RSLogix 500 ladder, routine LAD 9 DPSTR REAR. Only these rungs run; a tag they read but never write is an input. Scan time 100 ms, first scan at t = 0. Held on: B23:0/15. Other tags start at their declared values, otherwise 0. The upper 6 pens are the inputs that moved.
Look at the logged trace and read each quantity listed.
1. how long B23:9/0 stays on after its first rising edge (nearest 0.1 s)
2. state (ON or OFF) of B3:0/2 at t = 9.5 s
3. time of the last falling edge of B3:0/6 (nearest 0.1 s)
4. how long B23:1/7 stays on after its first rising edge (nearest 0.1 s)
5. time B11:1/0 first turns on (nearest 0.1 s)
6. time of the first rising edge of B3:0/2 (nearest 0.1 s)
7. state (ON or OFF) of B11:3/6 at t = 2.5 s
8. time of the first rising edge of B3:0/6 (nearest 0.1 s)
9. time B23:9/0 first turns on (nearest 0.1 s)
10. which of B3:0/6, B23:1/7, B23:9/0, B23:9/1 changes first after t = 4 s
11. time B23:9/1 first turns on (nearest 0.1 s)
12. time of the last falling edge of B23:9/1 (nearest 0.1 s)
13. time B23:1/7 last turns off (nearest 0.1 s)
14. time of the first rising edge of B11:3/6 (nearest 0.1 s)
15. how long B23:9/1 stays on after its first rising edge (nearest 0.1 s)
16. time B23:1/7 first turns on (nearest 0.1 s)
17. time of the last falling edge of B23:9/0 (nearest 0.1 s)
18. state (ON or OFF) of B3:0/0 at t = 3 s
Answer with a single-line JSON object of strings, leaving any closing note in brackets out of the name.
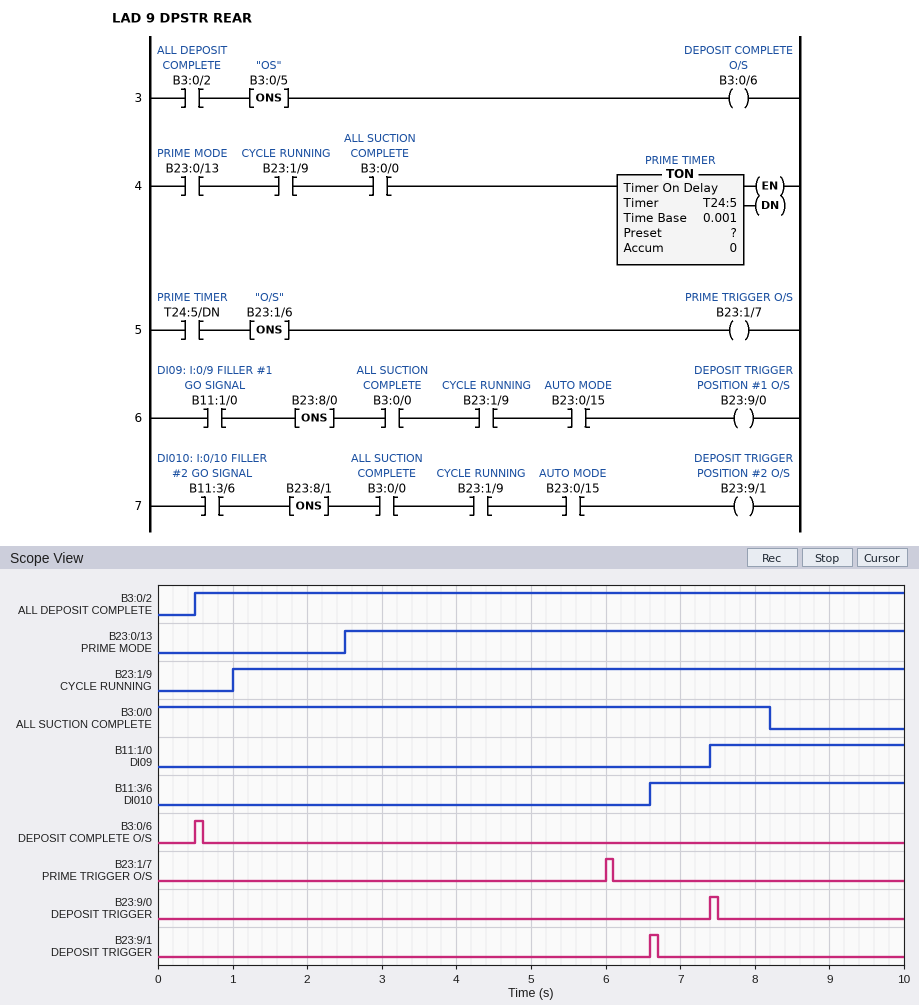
{"how long B23:9/0 stays on after its first rising edge": "0.1 s", "state (ON or OFF) of B3:0/2 at t = 9.5 s": "ON", "time of the last falling edge of B3:0/6": "0.6 s", "how long B23:1/7 stays on after its first rising edge": "0.1 s", "time B11:1/0 first turns on": "7.4 s", "time of the first rising edge of B3:0/2": "0.5 s", "state (ON or OFF) of B11:3/6 at t = 2.5 s": "OFF", "time of the first rising edge of B3:0/6": "0.5 s", "time B23:9/0 first turns on": "7.4 s", "which of B3:0/6, B23:1/7, B23:9/0, B23:9/1 changes first after t = 4 s": "B23:1/7", "time B23:9/1 first turns on": "6.6 s", "time of the last falling edge of B23:9/1": "6.7 s", "time B23:1/7 last turns off": "6.1 s", "time of the first rising edge of B11:3/6": "6.6 s", "how long B23:9/1 stays on after its first rising edge": "0.1 s", "time B23:1/7 first turns on": "6.0 s", "time of the last falling edge of B23:9/0": "7.5 s", "state (ON or OFF) of B3:0/0 at t = 3 s": "ON"}
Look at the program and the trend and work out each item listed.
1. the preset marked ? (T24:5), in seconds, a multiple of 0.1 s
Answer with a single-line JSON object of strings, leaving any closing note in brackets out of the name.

{"the preset marked ? (T24:5), in seconds, a multiple of 0.1 s": "3.5 s"}
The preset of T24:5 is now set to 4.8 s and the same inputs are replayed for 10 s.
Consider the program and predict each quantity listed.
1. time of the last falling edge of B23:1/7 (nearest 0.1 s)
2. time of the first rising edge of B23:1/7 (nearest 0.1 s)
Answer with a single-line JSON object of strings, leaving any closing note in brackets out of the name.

{"time of the last falling edge of B23:1/7": "7.4 s", "time of the first rising edge of B23:1/7": "7.3 s"}
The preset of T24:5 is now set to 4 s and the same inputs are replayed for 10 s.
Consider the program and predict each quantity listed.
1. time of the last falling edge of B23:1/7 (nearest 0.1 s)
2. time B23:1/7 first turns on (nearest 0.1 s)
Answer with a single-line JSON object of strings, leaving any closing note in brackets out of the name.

{"time of the last falling edge of B23:1/7": "6.6 s", "time B23:1/7 first turns on": "6.5 s"}
